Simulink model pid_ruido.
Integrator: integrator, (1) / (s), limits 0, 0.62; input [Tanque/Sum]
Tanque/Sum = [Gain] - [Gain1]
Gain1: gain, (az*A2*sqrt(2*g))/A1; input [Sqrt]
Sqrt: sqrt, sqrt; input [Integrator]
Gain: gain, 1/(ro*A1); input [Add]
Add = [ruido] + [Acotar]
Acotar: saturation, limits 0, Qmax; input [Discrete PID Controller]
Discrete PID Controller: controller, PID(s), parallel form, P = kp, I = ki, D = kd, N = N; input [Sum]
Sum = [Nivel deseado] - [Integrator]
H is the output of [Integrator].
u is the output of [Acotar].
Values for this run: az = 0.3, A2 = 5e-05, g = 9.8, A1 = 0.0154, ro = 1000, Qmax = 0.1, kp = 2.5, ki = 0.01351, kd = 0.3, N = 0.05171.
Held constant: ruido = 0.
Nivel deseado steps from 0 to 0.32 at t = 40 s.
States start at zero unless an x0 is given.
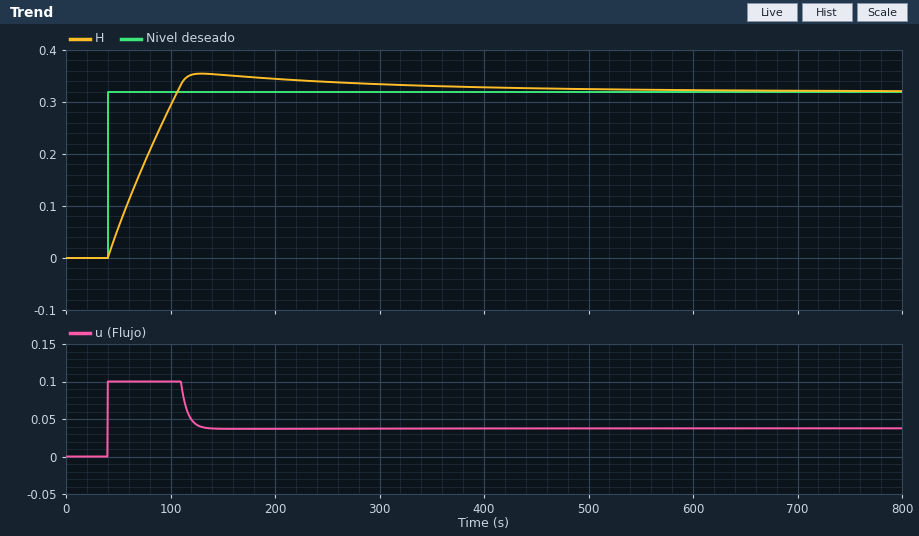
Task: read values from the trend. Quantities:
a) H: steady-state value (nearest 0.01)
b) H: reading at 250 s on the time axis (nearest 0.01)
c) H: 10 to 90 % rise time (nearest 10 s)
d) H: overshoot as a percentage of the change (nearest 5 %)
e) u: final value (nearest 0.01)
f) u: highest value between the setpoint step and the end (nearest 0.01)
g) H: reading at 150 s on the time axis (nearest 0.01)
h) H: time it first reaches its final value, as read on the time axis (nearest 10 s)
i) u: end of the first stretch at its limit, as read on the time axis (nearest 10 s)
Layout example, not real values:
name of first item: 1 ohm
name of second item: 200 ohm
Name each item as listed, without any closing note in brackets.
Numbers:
H: steady-state value: 0.32
H: reading at 250 s on the time axis: 0.34
H: 10 to 90 % rise time: 50 s
H: overshoot as a percentage of the change: 10 %
u: final value: 0.04
u: highest value between the setpoint step and the end: 0.10
H: reading at 150 s on the time axis: 0.35
H: time it first reaches its final value, as read on the time axis: 110 s
u: end of the first stretch at its limit, as read on the time axis: 110 s
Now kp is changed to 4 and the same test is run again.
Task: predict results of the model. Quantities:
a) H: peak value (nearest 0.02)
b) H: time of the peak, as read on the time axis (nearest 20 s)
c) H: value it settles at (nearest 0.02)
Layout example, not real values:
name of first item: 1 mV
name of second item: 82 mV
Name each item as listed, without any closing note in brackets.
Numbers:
H: peak value: 0.34
H: time of the peak, as read on the time axis: 120 s
H: value it settles at: 0.32
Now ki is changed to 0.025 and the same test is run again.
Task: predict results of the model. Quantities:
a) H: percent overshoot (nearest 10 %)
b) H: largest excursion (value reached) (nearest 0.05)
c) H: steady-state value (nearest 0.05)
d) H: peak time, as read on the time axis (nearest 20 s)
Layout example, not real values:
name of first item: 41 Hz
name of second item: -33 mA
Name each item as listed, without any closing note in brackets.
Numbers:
H: percent overshoot: 20 %
H: largest excursion (value reached): 0.40
H: steady-state value: 0.30
H: peak time, as read on the time axis: 140 s
